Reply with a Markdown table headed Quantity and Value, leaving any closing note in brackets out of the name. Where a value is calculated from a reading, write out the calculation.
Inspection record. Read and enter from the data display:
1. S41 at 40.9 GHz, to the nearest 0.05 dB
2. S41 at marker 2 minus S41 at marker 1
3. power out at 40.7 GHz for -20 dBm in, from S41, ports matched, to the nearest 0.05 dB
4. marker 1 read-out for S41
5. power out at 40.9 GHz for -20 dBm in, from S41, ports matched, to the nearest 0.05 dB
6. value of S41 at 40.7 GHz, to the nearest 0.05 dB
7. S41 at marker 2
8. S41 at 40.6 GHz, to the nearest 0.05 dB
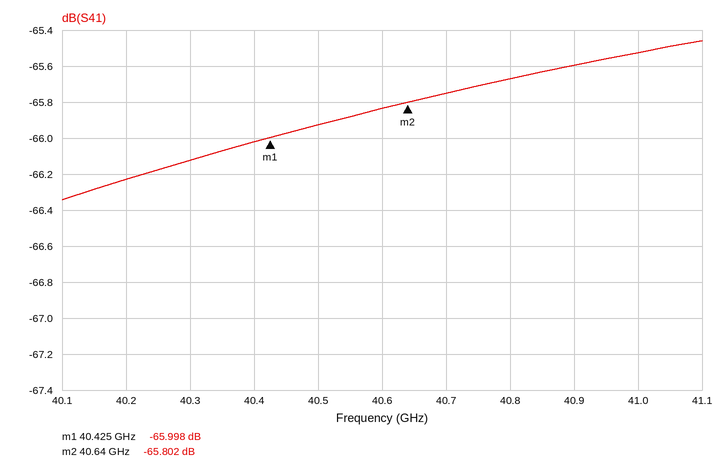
| Quantity | Value |
|---|---|
| S41 at 40.9 GHz, to the nearest 0.05 dB | -65.60 dB |
| S41 at marker 2 minus S41 at marker 1 | -65.802 − (-65.998) = 0.196 dB |
| power out at 40.7 GHz for -20 dBm in, from S41, ports matched, to the nearest 0.05 dB | -20 dBm + (-65.75 dB) = -85.75 dBm |
| marker 1 read-out for S41 | -65.998 dB |
| power out at 40.9 GHz for -20 dBm in, from S41, ports matched, to the nearest 0.05 dB | -20 dBm + (-65.60 dB) = -85.60 dBm |
| value of S41 at 40.7 GHz, to the nearest 0.05 dB | -65.75 dB |
| S41 at marker 2 | -65.802 dB |
| S41 at 40.6 GHz, to the nearest 0.05 dB | -65.85 dB |
